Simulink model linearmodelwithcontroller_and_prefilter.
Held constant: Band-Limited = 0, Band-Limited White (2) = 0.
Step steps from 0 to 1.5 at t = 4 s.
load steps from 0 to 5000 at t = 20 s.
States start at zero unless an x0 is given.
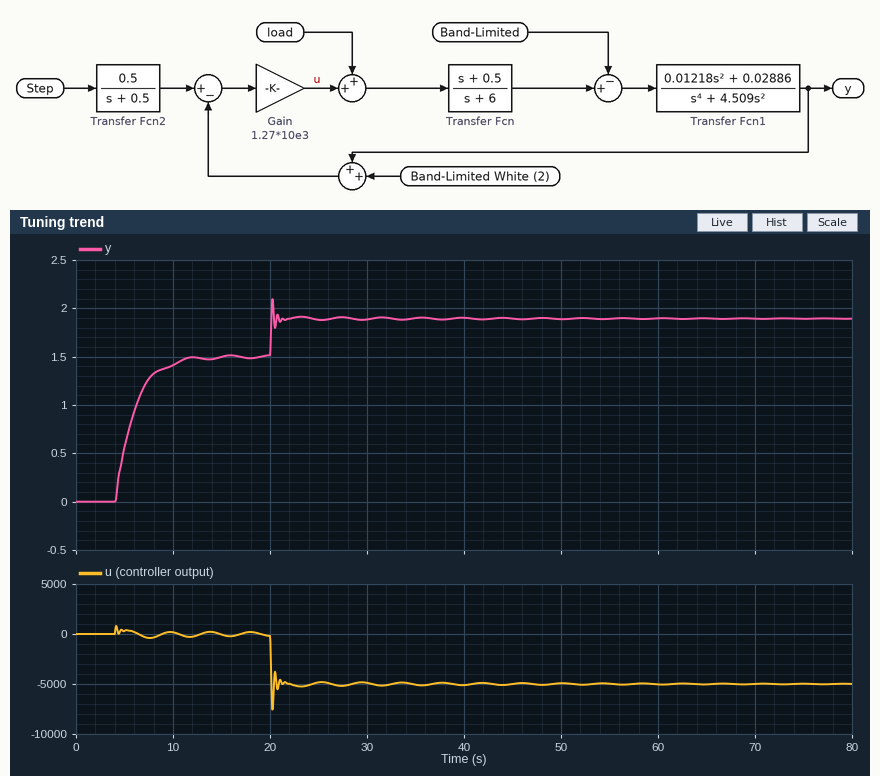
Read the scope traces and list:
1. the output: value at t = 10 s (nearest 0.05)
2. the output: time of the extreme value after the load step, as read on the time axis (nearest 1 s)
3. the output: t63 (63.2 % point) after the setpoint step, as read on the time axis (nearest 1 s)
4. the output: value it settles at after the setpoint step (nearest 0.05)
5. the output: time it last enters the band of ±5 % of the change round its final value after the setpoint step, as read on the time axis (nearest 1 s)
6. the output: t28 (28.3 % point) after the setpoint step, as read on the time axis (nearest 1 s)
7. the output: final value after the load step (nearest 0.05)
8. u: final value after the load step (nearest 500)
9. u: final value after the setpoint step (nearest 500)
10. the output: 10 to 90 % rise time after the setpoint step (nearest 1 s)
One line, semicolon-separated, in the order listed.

1.40; 20 s; 6 s; 1.50; 10 s; 5 s; 1.90; -5000; 0; 4 s
